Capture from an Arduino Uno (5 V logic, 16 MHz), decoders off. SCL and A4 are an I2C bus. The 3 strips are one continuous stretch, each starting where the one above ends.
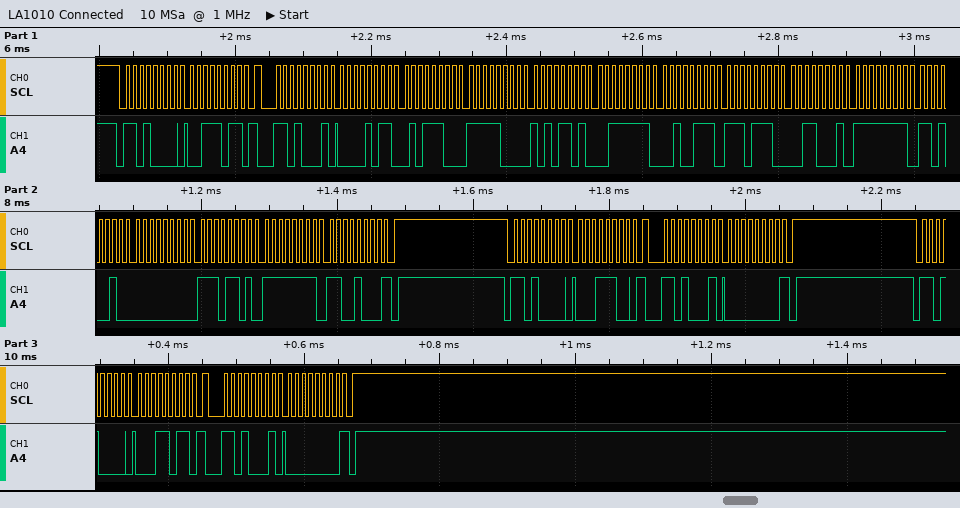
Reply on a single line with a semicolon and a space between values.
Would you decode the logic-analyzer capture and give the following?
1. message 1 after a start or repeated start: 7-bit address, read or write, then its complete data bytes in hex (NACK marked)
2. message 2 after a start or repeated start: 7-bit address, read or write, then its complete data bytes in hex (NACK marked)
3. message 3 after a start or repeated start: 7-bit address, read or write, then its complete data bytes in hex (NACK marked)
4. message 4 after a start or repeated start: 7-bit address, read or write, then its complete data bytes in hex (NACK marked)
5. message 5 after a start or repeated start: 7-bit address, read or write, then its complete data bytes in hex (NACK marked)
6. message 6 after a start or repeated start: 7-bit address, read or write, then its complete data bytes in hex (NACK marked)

0x68 write: 3B; 0x68 read: 0B 5C F8 AD 3F 27 EE 31 FF D2 00 ED FF C8 NACK; 0x68 write: 1C; 0x68 read: 00 NACK; 0x68 write: 1B; 0x68 read: 00 NACK
